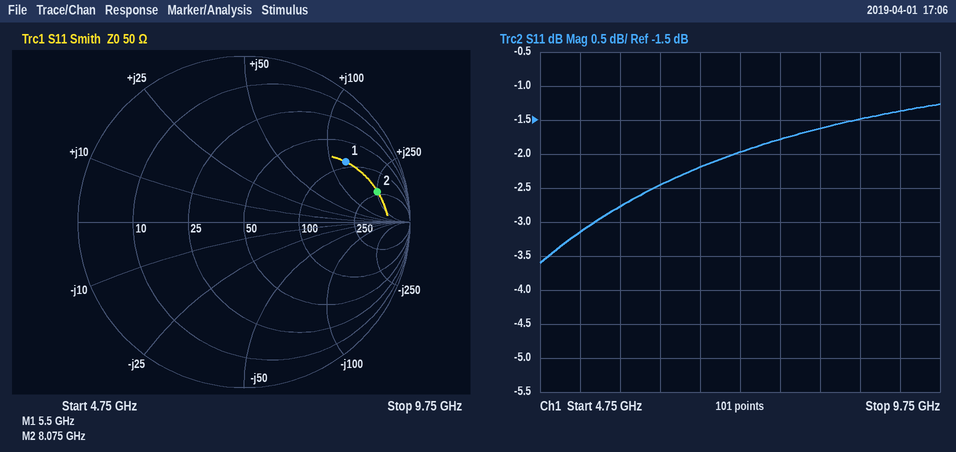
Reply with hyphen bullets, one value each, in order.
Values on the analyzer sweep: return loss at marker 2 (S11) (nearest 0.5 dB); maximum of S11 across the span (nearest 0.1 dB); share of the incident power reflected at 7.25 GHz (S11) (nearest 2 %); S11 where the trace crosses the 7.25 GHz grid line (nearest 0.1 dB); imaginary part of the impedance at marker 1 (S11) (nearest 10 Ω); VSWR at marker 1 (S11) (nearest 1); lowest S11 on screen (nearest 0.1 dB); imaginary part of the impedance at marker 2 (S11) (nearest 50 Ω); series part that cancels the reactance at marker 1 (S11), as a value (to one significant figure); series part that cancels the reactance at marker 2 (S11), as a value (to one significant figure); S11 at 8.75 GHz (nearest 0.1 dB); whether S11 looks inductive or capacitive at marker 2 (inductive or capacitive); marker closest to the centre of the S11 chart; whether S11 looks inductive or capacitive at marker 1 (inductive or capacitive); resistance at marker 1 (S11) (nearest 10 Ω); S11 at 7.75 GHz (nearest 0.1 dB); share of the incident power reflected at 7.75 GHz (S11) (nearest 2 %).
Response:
- 1.5 dB
- -1.3 dB
- 64 %
- -2.0 dB
- +130 Ω
- 6
- -3.6 dB
- +250 Ω
- 200 fF
- 80 fF
- -1.5 dB
- inductive
- marker 1
- inductive
- 90 Ω
- -1.8 dB
- 66 %
